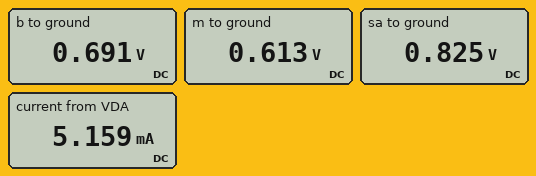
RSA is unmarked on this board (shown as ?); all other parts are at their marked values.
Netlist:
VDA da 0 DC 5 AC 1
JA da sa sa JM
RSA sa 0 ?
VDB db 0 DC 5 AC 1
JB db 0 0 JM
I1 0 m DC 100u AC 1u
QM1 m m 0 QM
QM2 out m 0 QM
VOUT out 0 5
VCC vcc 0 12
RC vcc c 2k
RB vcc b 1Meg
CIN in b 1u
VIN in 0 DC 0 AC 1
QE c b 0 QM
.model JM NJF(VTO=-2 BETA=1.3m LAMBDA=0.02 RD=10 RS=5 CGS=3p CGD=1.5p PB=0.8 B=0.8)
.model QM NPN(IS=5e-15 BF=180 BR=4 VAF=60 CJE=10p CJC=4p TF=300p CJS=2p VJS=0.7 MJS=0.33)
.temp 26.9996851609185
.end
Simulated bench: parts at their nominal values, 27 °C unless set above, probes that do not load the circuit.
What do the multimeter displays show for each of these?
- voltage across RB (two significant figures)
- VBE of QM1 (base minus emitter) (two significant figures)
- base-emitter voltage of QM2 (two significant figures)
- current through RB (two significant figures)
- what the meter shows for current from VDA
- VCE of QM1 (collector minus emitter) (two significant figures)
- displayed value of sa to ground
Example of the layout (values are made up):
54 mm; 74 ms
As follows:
11 V; 610 mV; 610 mV; 11 µA; 5.159 mA; 610 mV; 0.825 V
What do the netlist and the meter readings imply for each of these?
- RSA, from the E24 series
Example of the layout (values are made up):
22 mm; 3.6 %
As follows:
160 Ω
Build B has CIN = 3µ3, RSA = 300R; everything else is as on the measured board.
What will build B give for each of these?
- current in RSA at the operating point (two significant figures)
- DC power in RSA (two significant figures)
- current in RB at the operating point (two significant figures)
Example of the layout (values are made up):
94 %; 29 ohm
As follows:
5.1 mA; 7.8 mW; 11 µA
